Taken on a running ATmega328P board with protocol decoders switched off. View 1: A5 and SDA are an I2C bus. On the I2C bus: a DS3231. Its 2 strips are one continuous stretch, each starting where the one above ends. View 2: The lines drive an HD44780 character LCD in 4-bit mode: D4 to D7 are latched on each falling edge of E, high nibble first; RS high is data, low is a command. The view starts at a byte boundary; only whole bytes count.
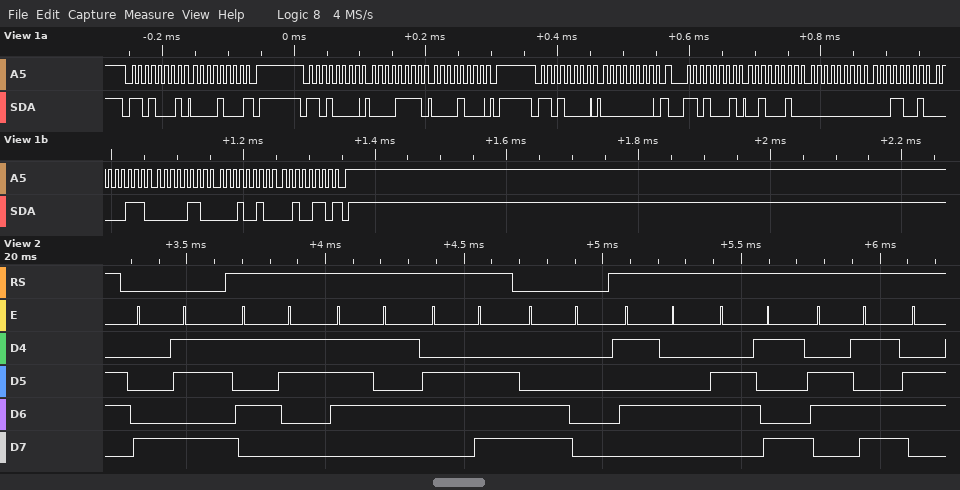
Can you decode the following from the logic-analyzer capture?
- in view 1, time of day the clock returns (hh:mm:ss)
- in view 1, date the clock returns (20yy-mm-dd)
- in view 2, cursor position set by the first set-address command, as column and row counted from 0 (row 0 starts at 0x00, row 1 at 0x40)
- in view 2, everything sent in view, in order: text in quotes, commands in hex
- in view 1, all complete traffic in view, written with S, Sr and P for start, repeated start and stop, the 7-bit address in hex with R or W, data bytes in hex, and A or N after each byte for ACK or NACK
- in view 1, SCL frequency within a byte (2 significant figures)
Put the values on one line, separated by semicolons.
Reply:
19:00:22; 2026-12-06; column 11, row 0; 0x8B "Sun" 0xC0 "Tim"; S 68R A 08 N P S 68W A 0F A 08 A P S 68W A 00 A Sr 68R A 22 A 00 A 19 A 07 A 06 A 12 A 26 N P; 100 kHz
